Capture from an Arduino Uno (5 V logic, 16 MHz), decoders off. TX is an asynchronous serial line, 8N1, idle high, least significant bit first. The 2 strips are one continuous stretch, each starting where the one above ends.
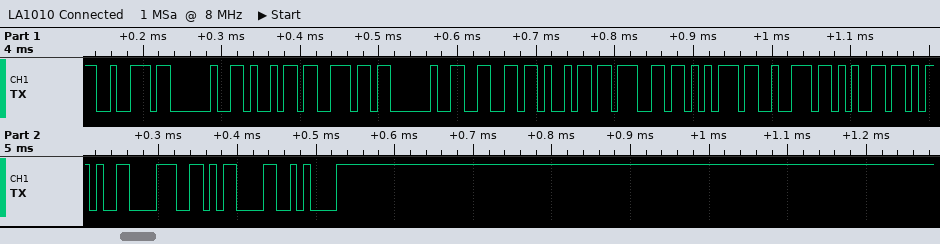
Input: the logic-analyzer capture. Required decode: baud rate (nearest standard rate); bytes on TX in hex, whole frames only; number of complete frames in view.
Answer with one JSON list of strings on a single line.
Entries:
["115200 baud", "72 20 69 6E 20 66 69 67 75 72 65 2D 38 0D 0A", "15"]
